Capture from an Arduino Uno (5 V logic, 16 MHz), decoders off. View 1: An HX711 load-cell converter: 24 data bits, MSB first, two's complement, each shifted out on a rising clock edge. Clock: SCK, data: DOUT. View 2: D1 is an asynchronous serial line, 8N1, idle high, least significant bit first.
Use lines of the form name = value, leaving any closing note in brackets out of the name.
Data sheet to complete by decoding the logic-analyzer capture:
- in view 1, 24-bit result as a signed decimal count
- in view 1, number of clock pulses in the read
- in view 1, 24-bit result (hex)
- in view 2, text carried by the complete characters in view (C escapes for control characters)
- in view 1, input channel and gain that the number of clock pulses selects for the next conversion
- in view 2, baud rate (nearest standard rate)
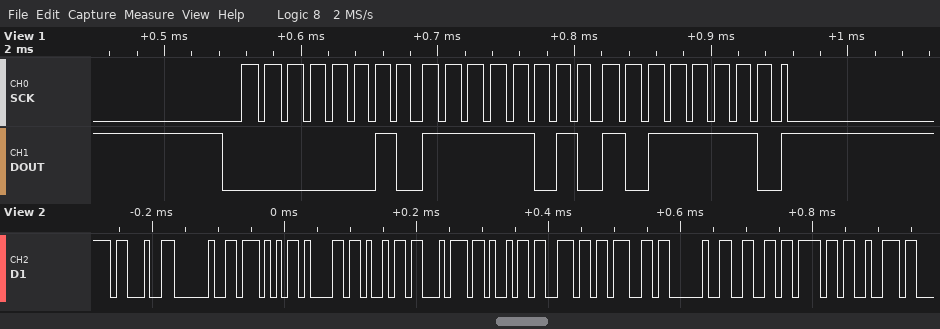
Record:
in view 1, 24-bit result as a signed decimal count = 195262
in view 1, number of clock pulses in the read = 25
in view 1, 24-bit result = 0x02FABE
in view 2, text carried by the complete characters in view = "# Waiting for"
in view 1, input channel and gain that the number of clock pulses selects for the next conversion = channel A, gain 128
in view 2, baud rate = 115200 baud
